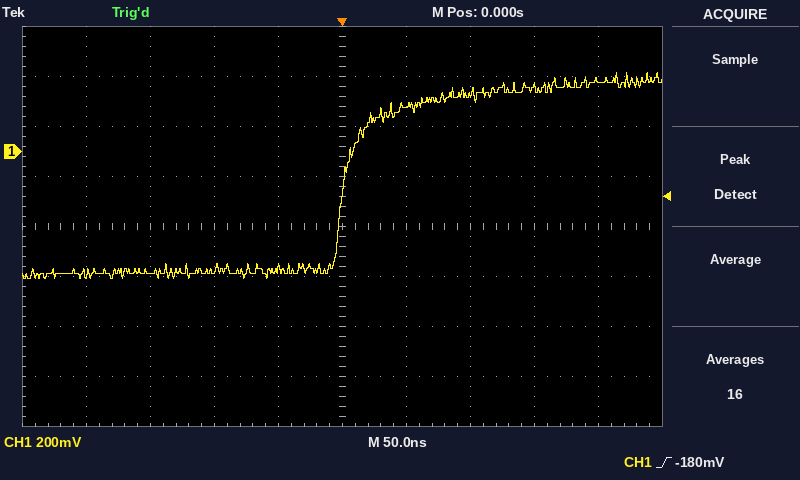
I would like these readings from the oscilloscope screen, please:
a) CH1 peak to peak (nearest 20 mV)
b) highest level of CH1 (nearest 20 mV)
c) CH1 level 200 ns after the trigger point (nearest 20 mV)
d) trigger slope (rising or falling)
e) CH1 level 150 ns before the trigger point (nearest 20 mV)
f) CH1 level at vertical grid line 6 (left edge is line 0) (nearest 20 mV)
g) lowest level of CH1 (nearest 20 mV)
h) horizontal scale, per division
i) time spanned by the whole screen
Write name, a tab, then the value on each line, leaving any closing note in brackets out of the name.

CH1 peak to peak	820 mV
highest level of CH1	320 mV
CH1 level 200 ns after the trigger point	280 mV
trigger slope	rising
CH1 level 150 ns before the trigger point	-480 mV
CH1 level at vertical grid line 6 (left edge is line 0)	180 mV
lowest level of CH1	-500 mV
horizontal scale, per division	50 ns
time spanned by the whole screen	500 ns
